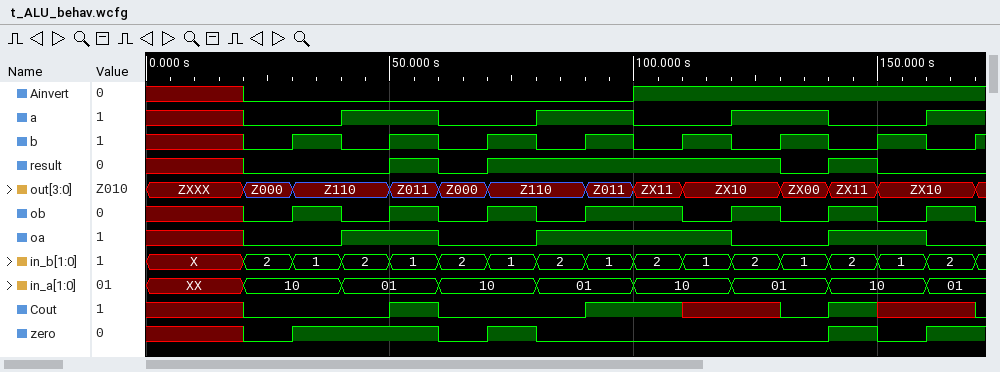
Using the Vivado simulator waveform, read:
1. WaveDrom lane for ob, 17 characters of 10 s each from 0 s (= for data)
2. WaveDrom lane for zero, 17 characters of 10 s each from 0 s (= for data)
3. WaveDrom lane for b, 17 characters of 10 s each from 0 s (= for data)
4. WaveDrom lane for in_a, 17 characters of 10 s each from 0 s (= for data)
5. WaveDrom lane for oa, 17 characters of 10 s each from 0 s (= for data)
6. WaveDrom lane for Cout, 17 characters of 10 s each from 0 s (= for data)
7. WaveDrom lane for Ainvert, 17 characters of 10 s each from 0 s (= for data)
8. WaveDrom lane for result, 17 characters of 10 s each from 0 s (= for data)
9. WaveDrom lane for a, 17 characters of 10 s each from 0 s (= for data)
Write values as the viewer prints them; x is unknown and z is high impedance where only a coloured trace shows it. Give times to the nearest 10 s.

{name: 'ob', wave: 'x.01010101.010101'}
{name: 'zero', wave: 'x.01..010.....101'}
{name: 'b', wave: 'x.010101010101010'}
{name: 'in_a', wave: 'x.=.=.=.=.=.=.=.=', data: '10 01 10 01 10 01 10 01'}
{name: 'oa', wave: 'x.0.1.0.1...0.1.0'}
{name: 'Cout', wave: 'x.0..10..1.x.01x.'}
{name: 'Ainvert', wave: 'x.0.......1......'}
{name: 'result', wave: 'x.0..101.....010.'}
{name: 'a', wave: 'x.0.1.0.1.0.1.0.1'}
